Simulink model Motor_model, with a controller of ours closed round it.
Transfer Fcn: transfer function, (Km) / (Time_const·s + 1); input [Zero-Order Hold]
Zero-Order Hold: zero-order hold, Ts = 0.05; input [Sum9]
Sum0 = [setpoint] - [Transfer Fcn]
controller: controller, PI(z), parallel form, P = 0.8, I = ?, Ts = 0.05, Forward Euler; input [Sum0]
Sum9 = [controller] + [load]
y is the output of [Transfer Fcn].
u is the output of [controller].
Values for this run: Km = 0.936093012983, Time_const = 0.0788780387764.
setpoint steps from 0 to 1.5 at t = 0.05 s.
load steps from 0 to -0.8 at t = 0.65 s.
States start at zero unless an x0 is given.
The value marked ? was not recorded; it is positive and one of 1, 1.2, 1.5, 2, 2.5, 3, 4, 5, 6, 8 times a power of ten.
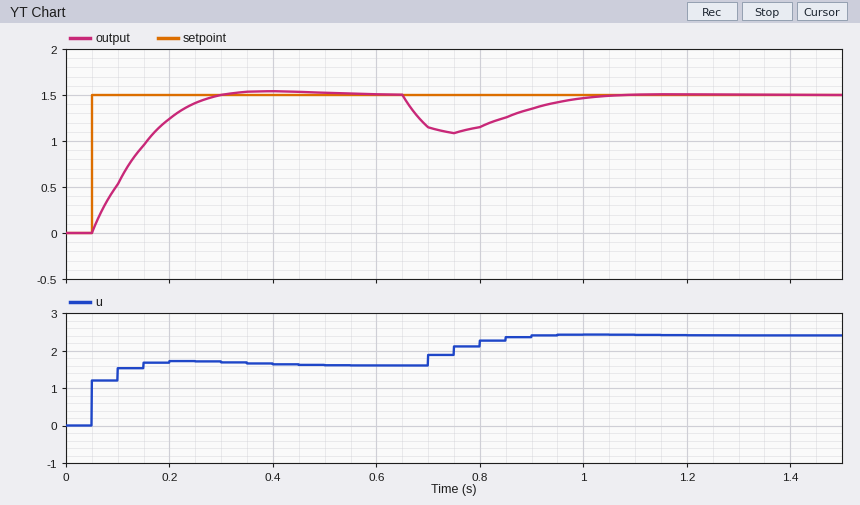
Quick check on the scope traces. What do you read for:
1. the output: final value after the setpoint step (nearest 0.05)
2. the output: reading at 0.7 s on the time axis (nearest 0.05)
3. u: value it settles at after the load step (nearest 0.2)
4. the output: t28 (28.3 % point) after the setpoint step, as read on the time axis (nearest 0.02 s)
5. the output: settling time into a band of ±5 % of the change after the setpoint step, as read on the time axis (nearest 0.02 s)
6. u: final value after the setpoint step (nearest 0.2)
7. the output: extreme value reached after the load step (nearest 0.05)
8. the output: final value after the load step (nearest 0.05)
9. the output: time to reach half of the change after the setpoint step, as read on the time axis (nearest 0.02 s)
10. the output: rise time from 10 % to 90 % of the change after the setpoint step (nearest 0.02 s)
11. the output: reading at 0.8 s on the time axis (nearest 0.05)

1.50
1.15
2.4
0.08 s
0.26 s
1.6
1.10
1.50
0.12 s
0.16 s
1.15
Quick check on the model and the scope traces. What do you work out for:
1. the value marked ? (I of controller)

10
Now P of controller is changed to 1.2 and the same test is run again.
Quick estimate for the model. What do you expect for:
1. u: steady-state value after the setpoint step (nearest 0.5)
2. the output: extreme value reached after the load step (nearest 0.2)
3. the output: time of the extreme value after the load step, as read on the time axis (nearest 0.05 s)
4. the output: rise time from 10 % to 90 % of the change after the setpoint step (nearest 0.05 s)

1.5
1.2
0.70 s
0.20 s
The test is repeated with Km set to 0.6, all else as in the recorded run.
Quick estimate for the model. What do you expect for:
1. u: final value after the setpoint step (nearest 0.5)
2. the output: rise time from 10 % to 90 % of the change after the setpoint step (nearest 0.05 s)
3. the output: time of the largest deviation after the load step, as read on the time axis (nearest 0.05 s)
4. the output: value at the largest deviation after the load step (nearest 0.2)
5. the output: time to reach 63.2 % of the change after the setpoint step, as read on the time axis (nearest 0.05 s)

2.5
0.30 s
0.75 s
1.2
0.20 s
